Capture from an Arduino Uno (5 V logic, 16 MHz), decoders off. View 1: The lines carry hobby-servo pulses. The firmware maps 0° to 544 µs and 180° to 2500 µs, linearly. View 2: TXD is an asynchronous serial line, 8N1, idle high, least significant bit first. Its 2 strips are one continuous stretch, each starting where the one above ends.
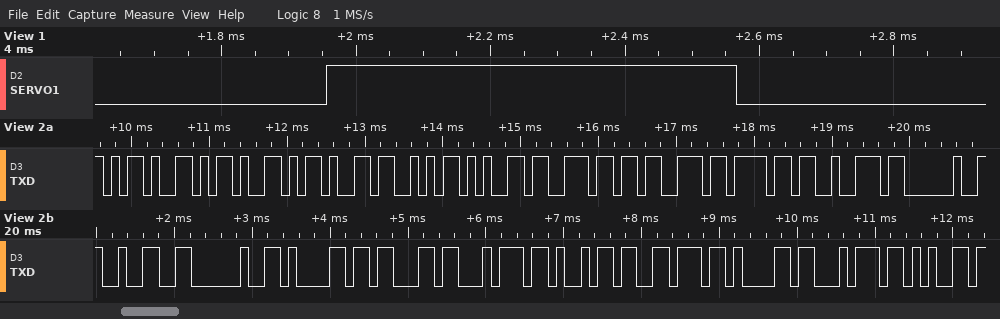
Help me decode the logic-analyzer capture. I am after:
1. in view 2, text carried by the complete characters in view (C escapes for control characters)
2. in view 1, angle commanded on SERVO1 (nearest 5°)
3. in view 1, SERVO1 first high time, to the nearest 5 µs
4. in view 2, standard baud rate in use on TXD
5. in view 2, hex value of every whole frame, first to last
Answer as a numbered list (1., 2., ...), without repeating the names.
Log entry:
1. "---Sensor 2 activate"
2. 5°
3. 610 µs
4. 9600 baud
5. 0x2D 0x2D 0x2D 0x53 0x65 0x6E 0x73 0x6F 0x72 0x20 0x32 0x20 0x61 0x63 0x74 0x69 0x76 0x61 0x74 0x65
